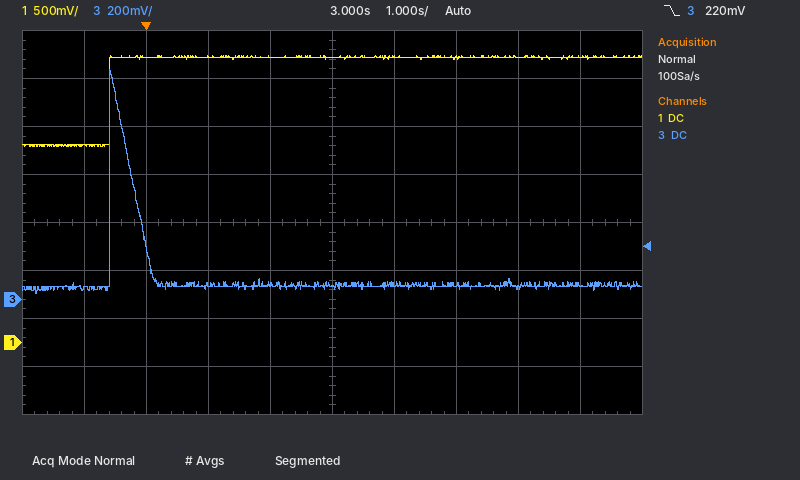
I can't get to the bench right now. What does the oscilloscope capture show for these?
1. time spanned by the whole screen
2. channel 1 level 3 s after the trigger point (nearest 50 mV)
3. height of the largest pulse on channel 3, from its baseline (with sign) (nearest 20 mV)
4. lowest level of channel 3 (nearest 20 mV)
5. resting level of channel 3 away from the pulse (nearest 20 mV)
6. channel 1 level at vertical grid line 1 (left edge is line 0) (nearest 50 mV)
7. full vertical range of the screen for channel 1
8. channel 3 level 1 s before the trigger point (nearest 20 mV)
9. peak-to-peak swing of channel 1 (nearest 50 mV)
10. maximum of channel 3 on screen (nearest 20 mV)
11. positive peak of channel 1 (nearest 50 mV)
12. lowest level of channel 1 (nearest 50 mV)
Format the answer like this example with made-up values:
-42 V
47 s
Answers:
10 s
2.95 V
+900 mV
20 mV
60 mV
2.05 V
4 V
40 mV
950 mV
960 mV
3.00 V
2.05 V
